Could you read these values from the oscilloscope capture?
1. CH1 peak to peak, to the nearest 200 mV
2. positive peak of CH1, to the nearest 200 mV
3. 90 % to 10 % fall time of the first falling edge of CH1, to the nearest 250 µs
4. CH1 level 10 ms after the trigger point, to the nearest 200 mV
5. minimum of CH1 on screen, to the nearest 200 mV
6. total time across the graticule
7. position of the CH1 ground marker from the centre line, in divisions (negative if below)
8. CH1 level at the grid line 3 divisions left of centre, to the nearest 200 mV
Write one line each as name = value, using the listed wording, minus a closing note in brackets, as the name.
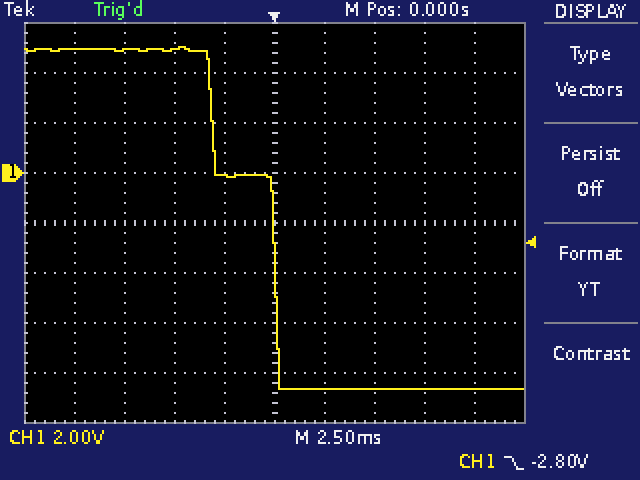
CH1 peak to peak, to the nearest 200 mV = 13.6 V
positive peak of CH1, to the nearest 200 mV = 5.0 V
90 % to 10 % fall time of the first falling edge of CH1, to the nearest 250 µs = 3.50 ms
CH1 level 10 ms after the trigger point, to the nearest 200 mV = -8.6 V
minimum of CH1 on screen, to the nearest 200 mV = -8.6 V
total time across the graticule = 25 ms
position of the CH1 ground marker from the centre line, in divisions = +1.0 div
CH1 level at the grid line 3 divisions left of centre, to the nearest 200 mV = 5.0 V
